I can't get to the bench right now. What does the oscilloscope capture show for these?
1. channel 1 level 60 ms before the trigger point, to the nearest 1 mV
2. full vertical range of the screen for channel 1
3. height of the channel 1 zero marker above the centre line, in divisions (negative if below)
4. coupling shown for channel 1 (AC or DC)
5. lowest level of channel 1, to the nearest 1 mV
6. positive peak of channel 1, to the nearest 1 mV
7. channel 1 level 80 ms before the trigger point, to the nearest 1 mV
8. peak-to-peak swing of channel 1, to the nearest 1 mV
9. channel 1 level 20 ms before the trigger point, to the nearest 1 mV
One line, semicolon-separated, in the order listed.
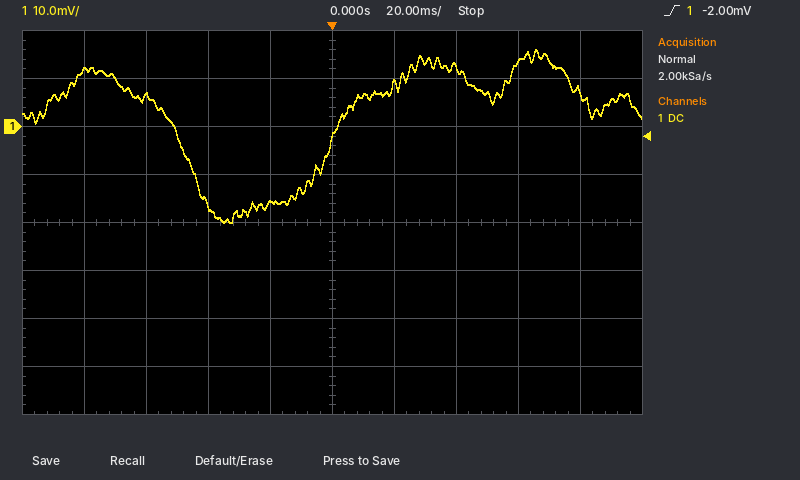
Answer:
6 mV; 80 mV; +2.0 div; DC; -20 mV; 16 mV; 12 mV; 36 mV; -16 mV
